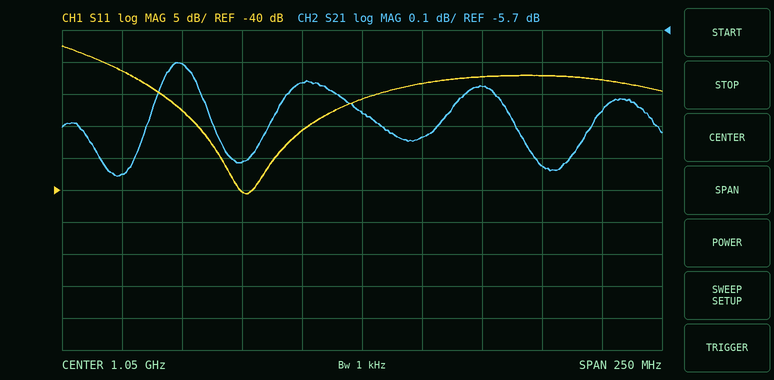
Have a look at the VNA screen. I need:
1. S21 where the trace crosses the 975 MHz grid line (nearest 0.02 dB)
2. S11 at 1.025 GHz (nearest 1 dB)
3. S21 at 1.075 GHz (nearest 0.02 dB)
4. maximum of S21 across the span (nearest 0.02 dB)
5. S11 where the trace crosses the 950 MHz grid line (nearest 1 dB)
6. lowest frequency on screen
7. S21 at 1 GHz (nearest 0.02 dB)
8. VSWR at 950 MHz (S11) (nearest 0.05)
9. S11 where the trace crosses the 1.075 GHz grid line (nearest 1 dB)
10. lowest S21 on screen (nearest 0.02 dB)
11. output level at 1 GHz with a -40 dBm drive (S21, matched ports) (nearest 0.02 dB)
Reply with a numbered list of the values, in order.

1. -5.80 dB
2. -31 dB
3. -6.04 dB
4. -5.80 dB
5. -21 dB
6. 925 MHz
7. -6.12 dB
8. 1.20
9. -23 dB
10. -6.16 dB
11. -46.12 dBm
